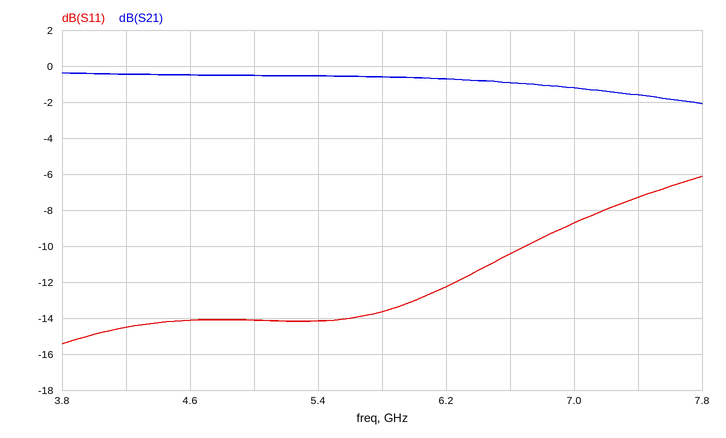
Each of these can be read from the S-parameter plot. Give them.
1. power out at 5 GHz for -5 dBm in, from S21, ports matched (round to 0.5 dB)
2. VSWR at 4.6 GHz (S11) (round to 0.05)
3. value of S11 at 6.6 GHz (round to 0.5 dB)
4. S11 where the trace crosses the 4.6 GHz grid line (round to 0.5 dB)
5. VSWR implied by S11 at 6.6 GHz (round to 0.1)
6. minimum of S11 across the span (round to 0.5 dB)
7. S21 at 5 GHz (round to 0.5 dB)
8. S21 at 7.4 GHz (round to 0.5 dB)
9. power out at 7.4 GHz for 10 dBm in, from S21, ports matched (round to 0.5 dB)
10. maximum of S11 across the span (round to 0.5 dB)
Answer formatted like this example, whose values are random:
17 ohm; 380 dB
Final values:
-5.5 dBm; 1.50; -10.5 dB; -14.0 dB; 1.9; -15.5 dB; -0.5 dB; -1.5 dB; 8.5 dBm; -6.0 dB
